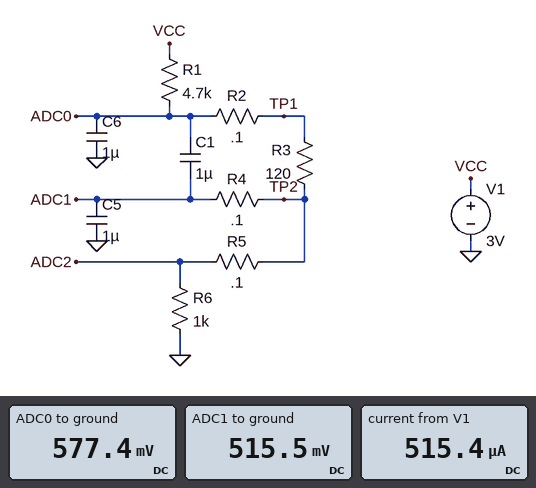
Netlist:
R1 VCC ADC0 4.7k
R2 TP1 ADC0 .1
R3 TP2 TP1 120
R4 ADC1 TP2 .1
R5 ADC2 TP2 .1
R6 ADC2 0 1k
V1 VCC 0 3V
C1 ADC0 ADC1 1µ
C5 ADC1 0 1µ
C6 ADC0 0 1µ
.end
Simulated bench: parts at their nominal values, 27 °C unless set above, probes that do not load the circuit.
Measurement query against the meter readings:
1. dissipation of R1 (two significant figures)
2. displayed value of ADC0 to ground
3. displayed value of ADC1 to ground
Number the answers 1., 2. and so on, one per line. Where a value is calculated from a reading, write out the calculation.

1. (3 V - 577.4 mV)^2 / 4.7 kΩ = 1.2 mW
2. 577.4 mV
3. 515.5 mV
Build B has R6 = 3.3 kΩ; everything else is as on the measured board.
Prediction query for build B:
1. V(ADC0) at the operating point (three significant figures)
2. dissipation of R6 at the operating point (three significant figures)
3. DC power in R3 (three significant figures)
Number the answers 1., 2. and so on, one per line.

1. 1.26 V
2. 450 µW
3. 16.4 µW
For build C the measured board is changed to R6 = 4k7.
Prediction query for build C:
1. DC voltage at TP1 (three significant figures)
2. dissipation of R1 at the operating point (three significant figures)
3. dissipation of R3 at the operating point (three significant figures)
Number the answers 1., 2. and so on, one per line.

1. 1.52 V
2. 467 µW
3. 11.9 µW
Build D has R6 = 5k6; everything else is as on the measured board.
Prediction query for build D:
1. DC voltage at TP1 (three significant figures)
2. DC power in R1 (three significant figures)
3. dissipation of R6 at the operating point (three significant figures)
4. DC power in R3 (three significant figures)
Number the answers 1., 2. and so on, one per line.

1. 1.65 V
2. 390 µW
3. 464 µW
4. 9.95 µW
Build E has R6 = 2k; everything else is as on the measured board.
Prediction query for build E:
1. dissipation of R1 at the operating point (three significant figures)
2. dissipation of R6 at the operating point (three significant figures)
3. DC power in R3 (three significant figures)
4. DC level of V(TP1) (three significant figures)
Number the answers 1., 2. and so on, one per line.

1. 909 µW
2. 387 µW
3. 23.2 µW
4. 933 mV
